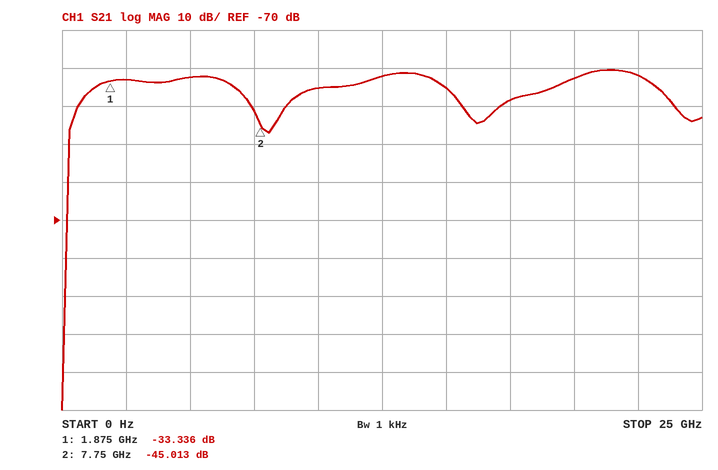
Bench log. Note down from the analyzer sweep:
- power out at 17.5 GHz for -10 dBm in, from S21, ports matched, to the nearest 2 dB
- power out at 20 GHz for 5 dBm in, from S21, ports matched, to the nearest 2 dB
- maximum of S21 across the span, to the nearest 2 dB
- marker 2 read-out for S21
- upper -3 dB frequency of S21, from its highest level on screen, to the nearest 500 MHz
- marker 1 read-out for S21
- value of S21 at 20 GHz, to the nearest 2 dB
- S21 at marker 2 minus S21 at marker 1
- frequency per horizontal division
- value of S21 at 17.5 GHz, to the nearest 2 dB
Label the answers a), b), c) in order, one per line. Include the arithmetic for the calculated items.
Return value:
a) -10 dBm + (-38 dB) = -48 dBm
b) 5 dBm + (-32 dB) = -28 dBm
c) -30 dB
d) -45.013 dB
e) 23.0 GHz
f) -33.336 dB
g) -32 dB
h) -45.013 − (-33.336) = -11.677 dB
i) 2.5 GHz
j) -38 dB
